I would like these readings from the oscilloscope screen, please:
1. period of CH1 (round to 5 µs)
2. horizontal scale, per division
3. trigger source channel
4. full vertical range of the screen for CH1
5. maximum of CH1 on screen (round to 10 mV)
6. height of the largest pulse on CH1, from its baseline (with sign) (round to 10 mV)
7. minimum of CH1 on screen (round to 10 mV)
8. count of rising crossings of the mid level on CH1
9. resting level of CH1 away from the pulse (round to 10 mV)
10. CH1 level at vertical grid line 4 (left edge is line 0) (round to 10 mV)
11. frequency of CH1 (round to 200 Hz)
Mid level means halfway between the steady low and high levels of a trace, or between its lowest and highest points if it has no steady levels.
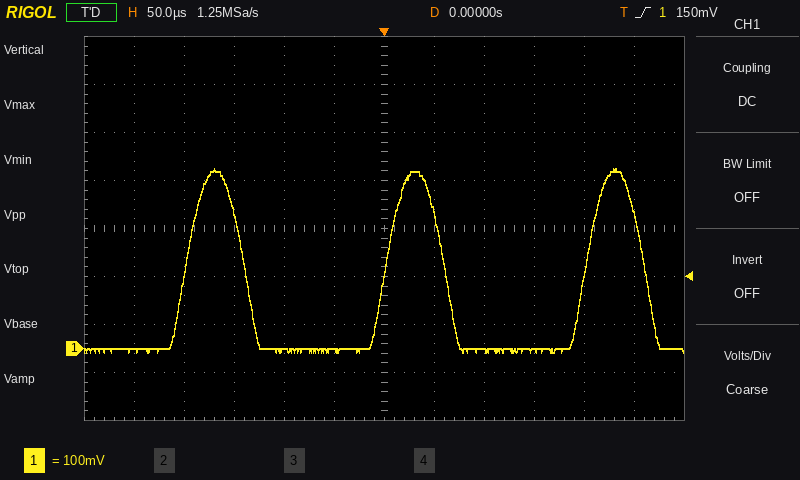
200 µs
50 µs
CH1
800 mV
380 mV
+380 mV
-10 mV
3
0 mV
0 mV
5.0 kHz
